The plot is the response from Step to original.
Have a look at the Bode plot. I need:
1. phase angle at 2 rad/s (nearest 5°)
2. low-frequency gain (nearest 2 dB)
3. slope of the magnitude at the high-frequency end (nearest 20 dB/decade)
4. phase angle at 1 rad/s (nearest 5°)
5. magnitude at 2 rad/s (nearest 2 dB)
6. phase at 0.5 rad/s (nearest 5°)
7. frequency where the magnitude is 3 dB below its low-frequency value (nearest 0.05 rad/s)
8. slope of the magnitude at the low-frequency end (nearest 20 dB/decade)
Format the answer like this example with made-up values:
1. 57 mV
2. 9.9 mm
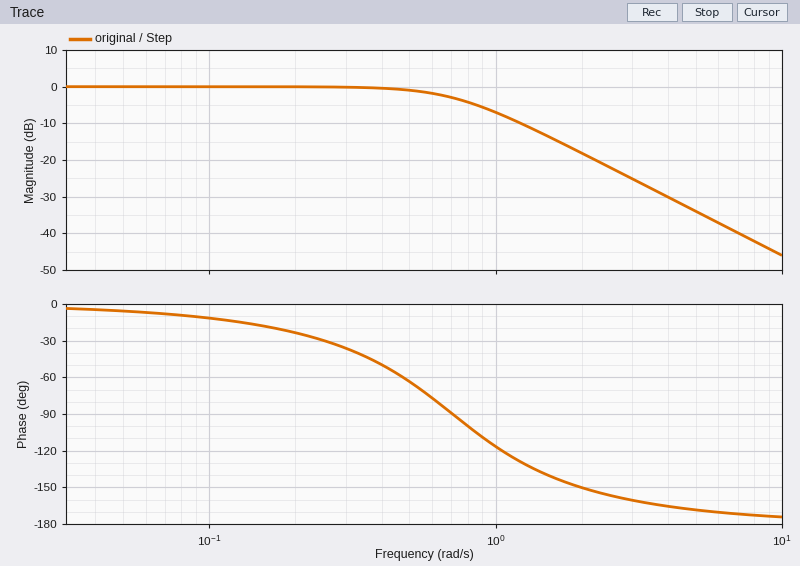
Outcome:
1. -150°
2. 0 dB
3. -40 dB/decade
4. -115°
5. -18 dB
6. -65°
7. 0.70 rad/s
8. 0 dB/decade
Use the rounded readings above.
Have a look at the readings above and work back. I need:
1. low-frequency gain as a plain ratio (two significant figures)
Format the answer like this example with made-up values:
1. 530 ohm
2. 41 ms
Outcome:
1. 1.0
